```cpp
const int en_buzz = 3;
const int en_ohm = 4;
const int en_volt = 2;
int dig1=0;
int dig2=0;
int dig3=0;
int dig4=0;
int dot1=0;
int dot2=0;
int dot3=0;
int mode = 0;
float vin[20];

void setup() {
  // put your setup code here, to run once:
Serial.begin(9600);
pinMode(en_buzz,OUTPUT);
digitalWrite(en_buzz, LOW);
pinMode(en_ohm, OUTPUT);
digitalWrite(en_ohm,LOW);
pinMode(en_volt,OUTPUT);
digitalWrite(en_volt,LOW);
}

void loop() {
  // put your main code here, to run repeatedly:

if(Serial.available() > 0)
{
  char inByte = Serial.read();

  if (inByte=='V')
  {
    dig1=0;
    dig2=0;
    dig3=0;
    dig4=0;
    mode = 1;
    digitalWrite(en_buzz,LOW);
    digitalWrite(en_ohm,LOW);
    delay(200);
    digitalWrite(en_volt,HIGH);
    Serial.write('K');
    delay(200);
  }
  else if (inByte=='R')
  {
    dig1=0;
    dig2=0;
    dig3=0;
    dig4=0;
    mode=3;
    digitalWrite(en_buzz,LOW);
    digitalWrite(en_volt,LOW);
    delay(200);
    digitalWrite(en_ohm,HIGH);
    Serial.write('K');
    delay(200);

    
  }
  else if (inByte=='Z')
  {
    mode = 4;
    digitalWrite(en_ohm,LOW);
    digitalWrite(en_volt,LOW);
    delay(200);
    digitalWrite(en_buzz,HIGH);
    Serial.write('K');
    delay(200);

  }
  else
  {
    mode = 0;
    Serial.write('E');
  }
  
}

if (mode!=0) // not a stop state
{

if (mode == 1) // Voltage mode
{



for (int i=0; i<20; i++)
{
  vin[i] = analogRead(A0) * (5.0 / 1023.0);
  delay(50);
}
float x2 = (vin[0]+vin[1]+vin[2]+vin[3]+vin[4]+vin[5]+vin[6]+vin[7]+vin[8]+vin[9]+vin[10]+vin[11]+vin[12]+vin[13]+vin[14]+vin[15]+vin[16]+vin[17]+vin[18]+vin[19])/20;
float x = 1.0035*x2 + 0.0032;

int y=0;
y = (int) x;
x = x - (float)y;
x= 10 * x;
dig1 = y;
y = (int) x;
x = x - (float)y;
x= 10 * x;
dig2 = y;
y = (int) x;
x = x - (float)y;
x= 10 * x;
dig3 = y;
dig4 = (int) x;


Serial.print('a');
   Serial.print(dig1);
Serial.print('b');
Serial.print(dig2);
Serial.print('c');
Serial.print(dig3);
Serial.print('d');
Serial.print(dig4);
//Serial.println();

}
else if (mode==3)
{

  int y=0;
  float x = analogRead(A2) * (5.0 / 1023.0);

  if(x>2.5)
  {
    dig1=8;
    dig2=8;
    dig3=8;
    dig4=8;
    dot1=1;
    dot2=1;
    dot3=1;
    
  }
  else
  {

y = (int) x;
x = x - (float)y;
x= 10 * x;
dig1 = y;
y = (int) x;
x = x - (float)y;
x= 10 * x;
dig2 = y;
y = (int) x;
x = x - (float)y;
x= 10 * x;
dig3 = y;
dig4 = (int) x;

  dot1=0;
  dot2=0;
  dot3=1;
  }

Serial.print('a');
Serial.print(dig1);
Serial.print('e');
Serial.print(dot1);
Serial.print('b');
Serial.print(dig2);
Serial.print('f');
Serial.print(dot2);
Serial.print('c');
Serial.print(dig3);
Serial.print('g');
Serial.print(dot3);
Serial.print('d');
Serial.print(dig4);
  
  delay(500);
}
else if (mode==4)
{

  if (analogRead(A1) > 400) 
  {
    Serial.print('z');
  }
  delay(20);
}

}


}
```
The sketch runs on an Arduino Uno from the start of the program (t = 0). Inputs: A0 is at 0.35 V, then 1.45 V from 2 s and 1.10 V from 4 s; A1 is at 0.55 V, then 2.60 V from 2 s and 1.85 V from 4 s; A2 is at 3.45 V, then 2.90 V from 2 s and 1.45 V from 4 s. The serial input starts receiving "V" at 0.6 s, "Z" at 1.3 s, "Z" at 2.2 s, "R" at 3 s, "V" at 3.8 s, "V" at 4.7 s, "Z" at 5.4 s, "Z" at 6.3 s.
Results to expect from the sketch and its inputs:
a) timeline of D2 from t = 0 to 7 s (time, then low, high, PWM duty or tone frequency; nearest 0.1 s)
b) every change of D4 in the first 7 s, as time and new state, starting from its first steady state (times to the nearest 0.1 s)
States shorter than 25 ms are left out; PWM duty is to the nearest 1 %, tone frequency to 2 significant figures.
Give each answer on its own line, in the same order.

0 s low; 0.8 s high; 2 s low; 4.1 s high; 6.7 s low
0 s low; 3.2 s high; 3.9 s low
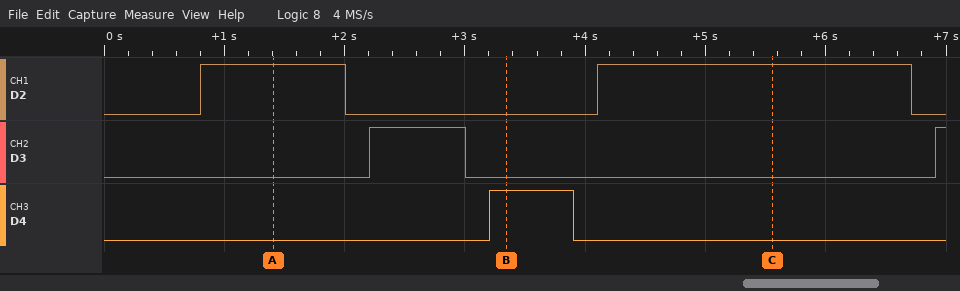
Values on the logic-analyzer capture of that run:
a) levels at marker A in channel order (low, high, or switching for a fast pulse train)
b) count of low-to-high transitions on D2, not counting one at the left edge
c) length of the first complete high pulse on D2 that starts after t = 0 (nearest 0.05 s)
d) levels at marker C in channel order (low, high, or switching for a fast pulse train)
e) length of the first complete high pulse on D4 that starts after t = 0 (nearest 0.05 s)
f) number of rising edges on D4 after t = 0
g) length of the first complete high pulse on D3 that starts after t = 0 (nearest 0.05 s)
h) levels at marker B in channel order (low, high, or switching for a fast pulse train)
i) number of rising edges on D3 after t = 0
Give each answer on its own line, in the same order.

D2 high, D3 low, D4 low
2
1.20 s
D2 high, D3 low, D4 low
0.70 s
1
0.80 s
D2 low, D3 low, D4 high
2
